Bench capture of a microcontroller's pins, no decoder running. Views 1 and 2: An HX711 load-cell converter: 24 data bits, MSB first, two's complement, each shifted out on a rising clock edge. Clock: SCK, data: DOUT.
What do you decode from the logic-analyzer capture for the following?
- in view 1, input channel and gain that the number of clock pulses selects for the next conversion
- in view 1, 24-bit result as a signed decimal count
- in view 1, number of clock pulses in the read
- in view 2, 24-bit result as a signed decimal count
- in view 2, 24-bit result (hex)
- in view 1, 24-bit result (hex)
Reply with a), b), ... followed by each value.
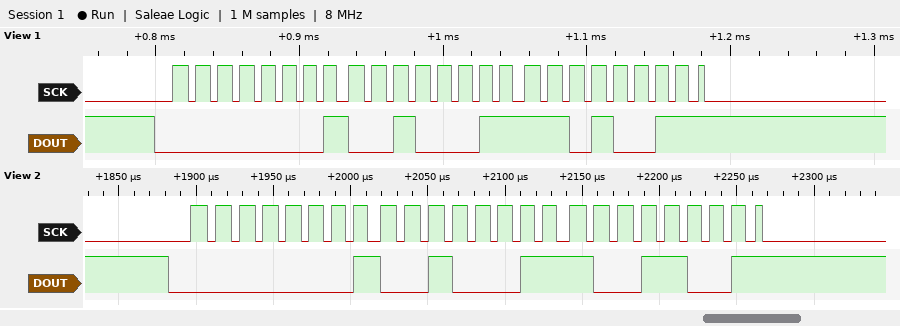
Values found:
a) channel A, gain 128
b) 74707
c) 25
d) 74649
e) 0x012399
f) 0x0123D3
